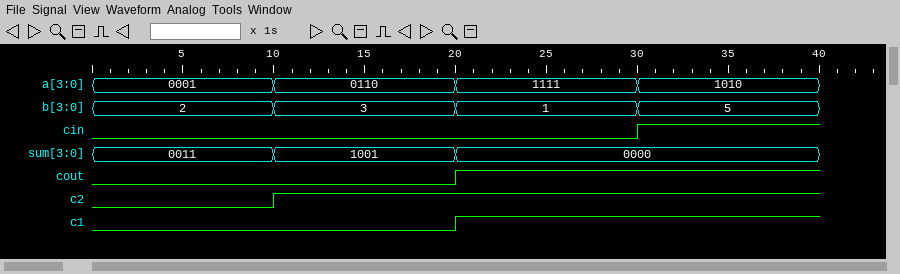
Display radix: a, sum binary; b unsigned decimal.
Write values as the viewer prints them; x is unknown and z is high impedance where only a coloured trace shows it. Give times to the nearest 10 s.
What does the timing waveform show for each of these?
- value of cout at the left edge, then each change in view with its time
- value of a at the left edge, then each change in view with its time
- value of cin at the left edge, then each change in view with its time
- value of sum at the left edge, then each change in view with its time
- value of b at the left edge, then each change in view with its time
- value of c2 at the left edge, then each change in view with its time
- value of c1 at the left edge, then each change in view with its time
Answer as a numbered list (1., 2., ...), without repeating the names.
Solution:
1. 0, 1 at 20 s
2. 0001, 0110 at 10 s, 1111 at 20 s, 1010 at 30 s
3. 0, 1 at 30 s
4. 0011, 1001 at 10 s, 0000 at 20 s
5. 2, 3 at 10 s, 1 at 20 s, 5 at 30 s
6. 0, 1 at 10 s
7. 0, 1 at 20 s
